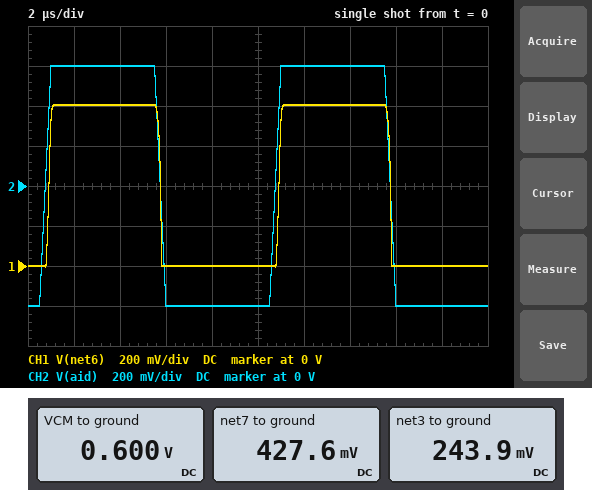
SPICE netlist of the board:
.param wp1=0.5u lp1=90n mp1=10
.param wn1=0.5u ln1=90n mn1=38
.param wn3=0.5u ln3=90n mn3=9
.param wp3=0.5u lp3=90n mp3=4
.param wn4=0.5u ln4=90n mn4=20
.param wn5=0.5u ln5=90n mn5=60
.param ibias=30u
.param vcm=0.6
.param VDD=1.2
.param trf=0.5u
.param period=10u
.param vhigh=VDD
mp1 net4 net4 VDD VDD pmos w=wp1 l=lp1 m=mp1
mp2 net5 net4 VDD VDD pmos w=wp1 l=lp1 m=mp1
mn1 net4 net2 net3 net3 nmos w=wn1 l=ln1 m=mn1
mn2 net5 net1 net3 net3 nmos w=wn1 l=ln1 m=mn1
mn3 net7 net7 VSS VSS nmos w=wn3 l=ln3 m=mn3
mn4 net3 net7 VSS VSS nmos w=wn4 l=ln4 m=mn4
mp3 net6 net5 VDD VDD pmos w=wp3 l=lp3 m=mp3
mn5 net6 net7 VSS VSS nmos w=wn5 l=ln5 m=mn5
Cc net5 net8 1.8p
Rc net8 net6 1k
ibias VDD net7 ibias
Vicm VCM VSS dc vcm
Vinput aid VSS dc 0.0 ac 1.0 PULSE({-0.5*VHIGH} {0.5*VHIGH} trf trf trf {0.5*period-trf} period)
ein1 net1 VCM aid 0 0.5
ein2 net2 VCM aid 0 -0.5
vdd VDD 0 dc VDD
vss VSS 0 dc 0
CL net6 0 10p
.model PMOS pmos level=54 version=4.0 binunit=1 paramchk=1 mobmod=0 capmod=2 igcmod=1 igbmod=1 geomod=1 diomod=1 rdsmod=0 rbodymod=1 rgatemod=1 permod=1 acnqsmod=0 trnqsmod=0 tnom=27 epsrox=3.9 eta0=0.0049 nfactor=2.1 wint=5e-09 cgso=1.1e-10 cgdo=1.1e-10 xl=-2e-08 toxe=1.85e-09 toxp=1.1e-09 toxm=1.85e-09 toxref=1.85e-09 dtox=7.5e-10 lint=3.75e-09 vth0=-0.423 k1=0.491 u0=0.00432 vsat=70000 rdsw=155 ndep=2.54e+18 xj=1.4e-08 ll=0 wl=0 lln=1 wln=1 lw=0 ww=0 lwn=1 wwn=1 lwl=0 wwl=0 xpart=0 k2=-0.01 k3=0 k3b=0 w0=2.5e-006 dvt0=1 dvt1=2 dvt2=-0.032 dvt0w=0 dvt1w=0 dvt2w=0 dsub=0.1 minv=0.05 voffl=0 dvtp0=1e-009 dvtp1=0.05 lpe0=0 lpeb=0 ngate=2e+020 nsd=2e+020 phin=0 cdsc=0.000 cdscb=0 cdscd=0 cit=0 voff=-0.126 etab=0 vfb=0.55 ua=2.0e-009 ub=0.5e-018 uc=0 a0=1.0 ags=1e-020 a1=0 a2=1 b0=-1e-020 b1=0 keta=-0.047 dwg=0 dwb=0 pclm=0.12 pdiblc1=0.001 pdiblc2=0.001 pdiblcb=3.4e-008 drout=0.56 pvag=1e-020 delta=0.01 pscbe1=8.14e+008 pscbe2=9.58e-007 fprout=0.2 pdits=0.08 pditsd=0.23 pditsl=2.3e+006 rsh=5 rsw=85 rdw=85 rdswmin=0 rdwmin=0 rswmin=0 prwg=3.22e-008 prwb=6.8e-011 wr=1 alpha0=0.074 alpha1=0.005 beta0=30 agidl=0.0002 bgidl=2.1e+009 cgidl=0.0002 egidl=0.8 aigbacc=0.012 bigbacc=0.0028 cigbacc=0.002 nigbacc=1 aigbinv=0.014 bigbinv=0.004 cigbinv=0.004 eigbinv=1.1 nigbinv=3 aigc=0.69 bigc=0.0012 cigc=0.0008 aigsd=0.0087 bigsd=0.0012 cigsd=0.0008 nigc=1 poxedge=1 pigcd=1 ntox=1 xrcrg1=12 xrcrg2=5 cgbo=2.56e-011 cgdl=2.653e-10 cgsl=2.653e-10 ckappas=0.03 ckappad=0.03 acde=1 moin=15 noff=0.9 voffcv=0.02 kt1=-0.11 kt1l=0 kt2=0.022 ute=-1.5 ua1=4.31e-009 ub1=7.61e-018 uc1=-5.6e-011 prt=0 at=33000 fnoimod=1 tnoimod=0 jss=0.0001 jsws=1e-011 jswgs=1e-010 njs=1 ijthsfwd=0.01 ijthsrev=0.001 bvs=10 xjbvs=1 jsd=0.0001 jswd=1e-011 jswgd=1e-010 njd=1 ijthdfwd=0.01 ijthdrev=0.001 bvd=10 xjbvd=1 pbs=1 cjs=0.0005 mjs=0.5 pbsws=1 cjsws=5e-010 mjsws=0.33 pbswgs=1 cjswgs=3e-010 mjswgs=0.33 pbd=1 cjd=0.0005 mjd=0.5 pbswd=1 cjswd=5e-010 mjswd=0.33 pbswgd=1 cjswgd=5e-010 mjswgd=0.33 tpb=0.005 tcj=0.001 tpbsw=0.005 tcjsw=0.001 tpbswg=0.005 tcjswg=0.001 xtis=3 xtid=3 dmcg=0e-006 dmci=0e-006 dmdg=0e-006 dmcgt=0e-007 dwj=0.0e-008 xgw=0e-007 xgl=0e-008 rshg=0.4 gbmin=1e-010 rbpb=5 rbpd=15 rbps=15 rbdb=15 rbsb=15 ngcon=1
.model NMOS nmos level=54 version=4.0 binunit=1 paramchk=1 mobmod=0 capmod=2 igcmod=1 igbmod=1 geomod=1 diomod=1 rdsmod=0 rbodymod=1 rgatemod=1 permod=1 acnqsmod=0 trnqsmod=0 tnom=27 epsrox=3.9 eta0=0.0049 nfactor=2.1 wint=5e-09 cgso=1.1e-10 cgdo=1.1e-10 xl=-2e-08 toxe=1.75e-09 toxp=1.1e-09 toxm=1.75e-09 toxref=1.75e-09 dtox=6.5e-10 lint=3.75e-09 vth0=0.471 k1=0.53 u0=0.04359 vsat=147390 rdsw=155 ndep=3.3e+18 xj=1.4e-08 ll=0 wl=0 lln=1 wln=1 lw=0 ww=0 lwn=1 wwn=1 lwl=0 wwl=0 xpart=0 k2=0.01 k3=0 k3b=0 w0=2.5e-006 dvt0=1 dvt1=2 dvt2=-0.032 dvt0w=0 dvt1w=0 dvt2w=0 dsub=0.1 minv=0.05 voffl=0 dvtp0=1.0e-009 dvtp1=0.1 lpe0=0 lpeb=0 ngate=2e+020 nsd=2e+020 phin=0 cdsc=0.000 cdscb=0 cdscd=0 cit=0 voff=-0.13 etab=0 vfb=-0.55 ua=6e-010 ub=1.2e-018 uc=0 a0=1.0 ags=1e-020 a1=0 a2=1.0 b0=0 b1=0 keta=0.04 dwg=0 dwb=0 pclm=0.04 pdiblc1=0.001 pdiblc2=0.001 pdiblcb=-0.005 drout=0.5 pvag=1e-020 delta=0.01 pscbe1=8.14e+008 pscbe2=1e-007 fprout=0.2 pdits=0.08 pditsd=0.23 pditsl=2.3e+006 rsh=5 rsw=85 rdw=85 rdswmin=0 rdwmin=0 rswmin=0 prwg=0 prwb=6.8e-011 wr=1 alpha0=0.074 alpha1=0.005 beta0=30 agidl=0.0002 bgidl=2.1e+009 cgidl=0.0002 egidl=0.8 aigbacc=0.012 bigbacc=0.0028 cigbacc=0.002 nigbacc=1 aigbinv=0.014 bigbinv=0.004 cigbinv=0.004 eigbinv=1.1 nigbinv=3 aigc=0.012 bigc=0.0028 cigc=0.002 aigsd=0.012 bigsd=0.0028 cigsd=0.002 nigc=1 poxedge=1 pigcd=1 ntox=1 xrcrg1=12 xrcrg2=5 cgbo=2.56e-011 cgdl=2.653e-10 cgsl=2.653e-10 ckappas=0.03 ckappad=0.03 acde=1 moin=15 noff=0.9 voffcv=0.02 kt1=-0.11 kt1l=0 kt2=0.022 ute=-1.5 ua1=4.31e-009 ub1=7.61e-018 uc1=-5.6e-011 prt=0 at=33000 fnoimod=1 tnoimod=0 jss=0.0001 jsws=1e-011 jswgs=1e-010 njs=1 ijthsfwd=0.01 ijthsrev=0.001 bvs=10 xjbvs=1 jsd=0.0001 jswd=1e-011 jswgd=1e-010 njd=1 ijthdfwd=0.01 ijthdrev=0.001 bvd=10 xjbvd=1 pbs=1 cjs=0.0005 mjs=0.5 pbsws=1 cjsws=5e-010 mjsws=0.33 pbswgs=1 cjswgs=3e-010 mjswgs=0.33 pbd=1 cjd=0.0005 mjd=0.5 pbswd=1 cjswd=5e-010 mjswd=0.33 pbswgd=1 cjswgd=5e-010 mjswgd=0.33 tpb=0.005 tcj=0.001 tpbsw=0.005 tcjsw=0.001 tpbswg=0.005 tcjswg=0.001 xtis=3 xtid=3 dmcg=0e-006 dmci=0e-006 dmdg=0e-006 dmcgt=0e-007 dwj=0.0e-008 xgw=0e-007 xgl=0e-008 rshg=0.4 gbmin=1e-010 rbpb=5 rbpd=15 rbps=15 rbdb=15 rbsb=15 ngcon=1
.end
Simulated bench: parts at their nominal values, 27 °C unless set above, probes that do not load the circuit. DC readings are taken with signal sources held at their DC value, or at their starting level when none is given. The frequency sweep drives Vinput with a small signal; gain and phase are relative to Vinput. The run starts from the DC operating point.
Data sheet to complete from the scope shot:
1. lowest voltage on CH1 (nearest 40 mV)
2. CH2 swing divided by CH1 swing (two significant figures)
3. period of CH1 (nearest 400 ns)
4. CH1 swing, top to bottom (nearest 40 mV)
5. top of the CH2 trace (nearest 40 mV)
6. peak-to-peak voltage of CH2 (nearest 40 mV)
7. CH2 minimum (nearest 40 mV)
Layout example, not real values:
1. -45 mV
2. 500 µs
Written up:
1. 0 V
2. 1.5
3. 10.0 µs
4. 800 mV
5. 600 mV
6. 1.20 V
7. -600 mV
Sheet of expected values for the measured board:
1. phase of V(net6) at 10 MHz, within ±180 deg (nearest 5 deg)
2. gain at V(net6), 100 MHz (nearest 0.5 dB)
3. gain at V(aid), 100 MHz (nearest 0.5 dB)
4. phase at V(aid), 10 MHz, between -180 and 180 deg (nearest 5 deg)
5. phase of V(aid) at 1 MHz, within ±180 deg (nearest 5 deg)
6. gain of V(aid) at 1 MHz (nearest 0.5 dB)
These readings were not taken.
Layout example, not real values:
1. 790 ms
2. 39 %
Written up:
1. -115 deg
2. -24.0 dB
3. 0 dB
4. 0 deg
5. 0 deg
6. 0 dB
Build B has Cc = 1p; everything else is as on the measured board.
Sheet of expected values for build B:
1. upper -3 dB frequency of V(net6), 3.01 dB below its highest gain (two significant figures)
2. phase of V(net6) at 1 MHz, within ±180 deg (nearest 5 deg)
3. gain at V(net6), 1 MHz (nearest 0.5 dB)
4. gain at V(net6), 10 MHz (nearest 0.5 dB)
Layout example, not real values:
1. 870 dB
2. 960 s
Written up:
1. 2.9 MHz
2. -20 deg
3. 1.0 dB
4. -9.5 dB
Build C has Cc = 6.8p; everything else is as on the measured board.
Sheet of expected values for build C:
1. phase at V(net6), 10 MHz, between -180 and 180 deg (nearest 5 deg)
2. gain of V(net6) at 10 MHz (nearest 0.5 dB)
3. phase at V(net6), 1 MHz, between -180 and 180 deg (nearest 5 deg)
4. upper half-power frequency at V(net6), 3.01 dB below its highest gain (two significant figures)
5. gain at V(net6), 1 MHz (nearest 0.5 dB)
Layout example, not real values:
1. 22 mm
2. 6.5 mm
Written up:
1. -160 deg
2. -19.0 dB
3. -80 deg
4. 430 kHz
5. -6.5 dB
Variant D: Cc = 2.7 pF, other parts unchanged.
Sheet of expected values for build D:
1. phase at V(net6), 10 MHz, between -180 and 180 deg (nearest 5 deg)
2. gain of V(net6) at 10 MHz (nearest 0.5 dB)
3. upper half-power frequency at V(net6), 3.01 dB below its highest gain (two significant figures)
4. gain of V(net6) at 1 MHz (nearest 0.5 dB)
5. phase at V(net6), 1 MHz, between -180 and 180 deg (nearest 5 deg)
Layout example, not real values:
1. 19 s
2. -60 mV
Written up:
1. -130 deg
2. -16.0 dB
3. 1.1 MHz
4. -1.5 dB
5. -50 deg
